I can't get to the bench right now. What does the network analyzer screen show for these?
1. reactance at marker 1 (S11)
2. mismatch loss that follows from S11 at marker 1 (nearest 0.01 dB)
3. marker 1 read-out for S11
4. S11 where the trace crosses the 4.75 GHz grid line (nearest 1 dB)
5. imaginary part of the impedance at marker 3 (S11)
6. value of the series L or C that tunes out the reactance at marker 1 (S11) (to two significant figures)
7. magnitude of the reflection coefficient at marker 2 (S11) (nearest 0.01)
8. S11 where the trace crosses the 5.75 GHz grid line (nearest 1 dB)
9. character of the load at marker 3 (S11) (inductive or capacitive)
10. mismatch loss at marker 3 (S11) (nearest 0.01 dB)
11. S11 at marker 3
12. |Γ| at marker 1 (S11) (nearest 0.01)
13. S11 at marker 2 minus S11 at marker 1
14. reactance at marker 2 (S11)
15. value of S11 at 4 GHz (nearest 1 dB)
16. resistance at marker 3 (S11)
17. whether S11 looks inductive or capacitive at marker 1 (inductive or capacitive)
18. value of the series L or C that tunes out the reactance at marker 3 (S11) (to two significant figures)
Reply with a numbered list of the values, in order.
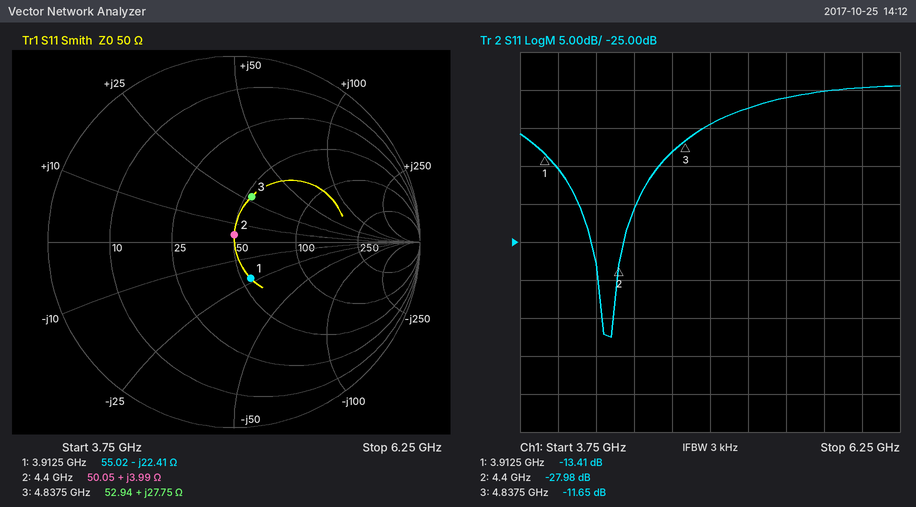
1. -22.41 Ω
2. 0.20 dB
3. -13.41 dB
4. -13 dB
5. +27.75 Ω
6. 910 pH
7. 0.04
8. -5 dB
9. inductive
10. 0.31 dB
11. -11.65 dB
12. 0.21
13. -14.57 dB
14. +3.99 Ω
15. -15 dB
16. 52.94 Ω
17. capacitive
18. 1.2 pF
